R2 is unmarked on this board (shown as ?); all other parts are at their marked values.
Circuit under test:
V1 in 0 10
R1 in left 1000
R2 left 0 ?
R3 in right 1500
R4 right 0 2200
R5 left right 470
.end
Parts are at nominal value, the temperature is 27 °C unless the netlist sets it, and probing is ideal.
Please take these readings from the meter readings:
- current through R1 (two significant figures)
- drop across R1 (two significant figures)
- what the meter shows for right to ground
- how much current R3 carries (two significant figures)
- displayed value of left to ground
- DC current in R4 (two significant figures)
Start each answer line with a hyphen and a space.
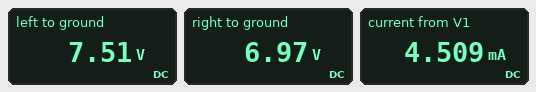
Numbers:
- 2.5 mA
- 2.5 V
- 6.97 V
- 2.0 mA
- 7.51 V
- 3.2 mA
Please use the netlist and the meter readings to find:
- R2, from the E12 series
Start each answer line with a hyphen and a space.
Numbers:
- 5.6 kΩ
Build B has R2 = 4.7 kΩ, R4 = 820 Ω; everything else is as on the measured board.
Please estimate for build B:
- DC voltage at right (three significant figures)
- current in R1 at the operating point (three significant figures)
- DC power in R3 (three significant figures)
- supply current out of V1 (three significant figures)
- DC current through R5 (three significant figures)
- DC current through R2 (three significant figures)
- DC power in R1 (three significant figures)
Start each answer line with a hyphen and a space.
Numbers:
- 4.90 V
- 3.88 mA
- 17.3 mW
- 7.28 mA
- 2.58 mA
- 1.30 mA
- 15.1 mW
